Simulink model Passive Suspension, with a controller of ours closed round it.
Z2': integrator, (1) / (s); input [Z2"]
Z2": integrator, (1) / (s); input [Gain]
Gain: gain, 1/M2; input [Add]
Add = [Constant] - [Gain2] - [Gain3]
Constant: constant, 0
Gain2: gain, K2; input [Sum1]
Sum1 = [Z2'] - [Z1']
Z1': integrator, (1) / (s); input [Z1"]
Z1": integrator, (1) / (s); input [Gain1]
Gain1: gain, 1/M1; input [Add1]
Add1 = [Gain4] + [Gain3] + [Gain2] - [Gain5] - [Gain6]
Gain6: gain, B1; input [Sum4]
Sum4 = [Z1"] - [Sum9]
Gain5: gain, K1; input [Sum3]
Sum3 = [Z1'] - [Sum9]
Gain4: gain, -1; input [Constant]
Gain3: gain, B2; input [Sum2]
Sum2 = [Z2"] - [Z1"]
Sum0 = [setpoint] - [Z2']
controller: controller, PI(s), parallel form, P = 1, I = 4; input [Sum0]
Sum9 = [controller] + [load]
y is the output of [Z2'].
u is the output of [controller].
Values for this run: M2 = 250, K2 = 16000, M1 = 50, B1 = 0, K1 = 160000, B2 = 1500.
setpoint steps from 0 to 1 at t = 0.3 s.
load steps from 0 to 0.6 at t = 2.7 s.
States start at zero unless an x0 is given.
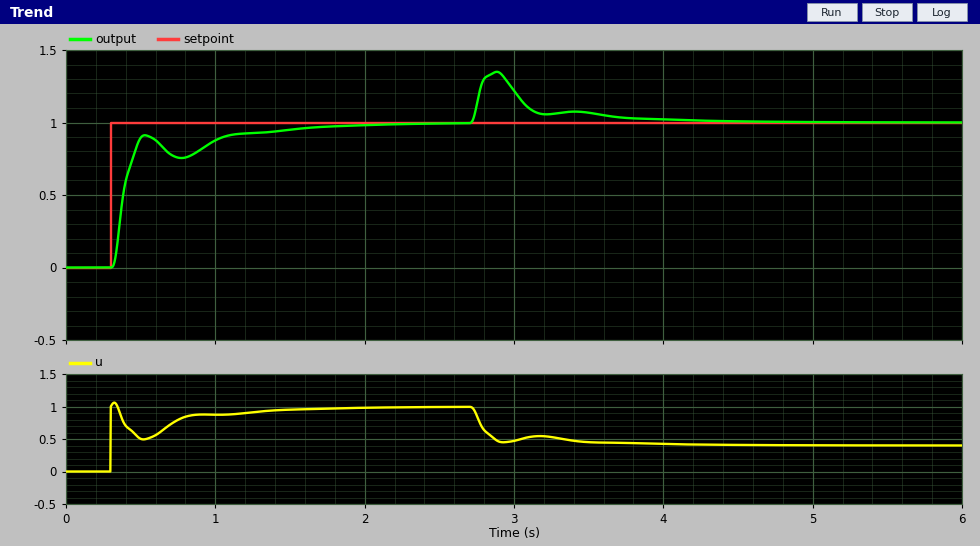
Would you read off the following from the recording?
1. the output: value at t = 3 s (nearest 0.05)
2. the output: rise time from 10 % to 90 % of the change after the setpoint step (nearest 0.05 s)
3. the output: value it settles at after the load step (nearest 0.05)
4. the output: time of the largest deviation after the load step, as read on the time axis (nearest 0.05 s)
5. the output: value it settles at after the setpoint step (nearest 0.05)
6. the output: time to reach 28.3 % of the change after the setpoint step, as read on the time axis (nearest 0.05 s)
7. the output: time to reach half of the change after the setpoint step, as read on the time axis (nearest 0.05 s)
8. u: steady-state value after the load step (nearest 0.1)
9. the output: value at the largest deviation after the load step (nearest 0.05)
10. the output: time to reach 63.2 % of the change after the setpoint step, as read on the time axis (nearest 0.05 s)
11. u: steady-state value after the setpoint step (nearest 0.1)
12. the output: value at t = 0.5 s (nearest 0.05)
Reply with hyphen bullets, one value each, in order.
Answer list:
- 1.20
- 0.15 s
- 1.00
- 2.90 s
- 1.00
- 0.35 s
- 0.40 s
- 0.4
- 1.35
- 0.40 s
- 1.0
- 0.90
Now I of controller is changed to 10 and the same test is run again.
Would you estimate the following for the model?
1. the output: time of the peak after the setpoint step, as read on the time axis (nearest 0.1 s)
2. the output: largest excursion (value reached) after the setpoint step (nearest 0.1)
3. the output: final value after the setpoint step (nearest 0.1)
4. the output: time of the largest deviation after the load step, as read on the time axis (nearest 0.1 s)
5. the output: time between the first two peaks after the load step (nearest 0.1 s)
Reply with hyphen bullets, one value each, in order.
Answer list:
- 0.5 s
- 1.2
- 1.0
- 2.8 s
- 0.5 s
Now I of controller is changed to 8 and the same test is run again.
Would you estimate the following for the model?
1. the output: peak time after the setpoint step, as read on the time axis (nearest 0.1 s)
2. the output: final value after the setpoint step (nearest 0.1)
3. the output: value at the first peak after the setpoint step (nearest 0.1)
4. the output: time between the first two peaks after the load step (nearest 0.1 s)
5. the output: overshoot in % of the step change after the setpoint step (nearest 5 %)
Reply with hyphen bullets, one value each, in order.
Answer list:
- 0.5 s
- 1.0
- 1.1
- 0.5 s
- 10 %
